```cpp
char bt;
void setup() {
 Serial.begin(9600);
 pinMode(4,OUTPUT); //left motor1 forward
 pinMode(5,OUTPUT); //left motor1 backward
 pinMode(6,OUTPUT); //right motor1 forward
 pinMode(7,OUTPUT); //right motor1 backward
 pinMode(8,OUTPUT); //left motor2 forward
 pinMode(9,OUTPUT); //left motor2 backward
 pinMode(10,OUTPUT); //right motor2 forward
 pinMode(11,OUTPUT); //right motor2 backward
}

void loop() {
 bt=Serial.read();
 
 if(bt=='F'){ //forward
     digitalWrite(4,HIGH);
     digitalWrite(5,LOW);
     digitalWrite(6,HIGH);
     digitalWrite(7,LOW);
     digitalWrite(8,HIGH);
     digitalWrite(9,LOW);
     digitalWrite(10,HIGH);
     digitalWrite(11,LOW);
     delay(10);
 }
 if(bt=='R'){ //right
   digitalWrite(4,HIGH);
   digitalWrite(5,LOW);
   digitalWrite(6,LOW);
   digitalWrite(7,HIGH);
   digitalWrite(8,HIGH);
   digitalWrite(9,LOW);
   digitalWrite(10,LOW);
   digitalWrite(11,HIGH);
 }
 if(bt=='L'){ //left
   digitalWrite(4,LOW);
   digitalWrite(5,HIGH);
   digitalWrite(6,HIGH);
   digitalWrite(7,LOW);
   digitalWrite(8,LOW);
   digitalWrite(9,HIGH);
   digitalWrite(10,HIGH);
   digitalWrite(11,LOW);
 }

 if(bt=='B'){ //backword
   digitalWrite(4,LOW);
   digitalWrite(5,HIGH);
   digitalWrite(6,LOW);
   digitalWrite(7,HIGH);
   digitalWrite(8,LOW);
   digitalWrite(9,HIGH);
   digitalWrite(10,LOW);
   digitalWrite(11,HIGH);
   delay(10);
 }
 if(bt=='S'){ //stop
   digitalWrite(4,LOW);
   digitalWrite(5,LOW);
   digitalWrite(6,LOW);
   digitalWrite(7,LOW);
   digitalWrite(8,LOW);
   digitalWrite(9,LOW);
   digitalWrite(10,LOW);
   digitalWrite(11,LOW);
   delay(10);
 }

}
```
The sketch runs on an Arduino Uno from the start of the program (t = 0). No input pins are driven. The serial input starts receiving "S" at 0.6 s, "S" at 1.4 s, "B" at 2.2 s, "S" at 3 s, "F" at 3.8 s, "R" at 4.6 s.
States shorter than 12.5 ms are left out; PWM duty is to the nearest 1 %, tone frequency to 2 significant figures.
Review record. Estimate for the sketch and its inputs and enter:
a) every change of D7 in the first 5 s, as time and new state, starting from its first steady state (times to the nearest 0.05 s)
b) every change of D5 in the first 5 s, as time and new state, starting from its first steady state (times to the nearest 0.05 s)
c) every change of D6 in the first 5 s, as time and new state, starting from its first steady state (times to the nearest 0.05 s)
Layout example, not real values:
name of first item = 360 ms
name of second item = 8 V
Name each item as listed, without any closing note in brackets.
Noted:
every change of D7 in the first 5 s, as time and new state, starting from its first steady state = 0 s low; 2.2 s high; 3 s low; 4.6 s high
every change of D5 in the first 5 s, as time and new state, starting from its first steady state = 0 s low; 2.2 s high; 3 s low
every change of D6 in the first 5 s, as time and new state, starting from its first steady state = 0 s low; 3.8 s high; 4.6 s low
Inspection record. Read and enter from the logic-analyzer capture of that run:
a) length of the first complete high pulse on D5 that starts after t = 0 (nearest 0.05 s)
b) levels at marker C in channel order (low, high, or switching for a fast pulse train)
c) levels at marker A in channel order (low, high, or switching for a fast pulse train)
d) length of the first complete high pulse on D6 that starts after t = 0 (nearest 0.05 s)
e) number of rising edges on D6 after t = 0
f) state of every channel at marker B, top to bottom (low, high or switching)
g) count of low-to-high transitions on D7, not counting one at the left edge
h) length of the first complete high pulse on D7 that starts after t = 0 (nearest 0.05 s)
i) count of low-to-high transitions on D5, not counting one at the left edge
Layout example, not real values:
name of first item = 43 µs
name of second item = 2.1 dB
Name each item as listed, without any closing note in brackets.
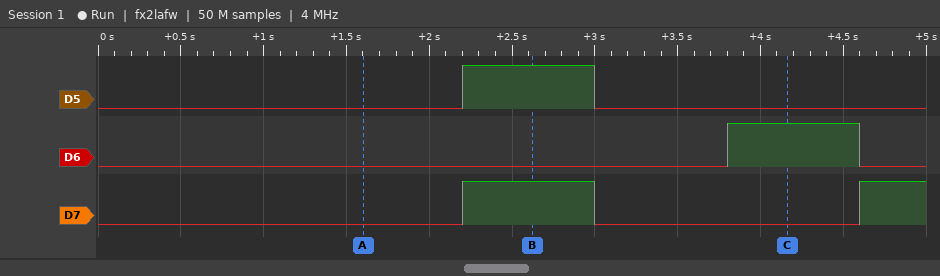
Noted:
length of the first complete high pulse on D5 that starts after t = 0 = 0.80 s
levels at marker C in channel order = D5 low, D6 high, D7 low
levels at marker A in channel order = D5 low, D6 low, D7 low
length of the first complete high pulse on D6 that starts after t = 0 = 0.80 s
number of rising edges on D6 after t = 0 = 1
state of every channel at marker B, top to bottom = D5 high, D6 low, D7 high
count of low-to-high transitions on D7, not counting one at the left edge = 2
length of the first complete high pulse on D7 that starts after t = 0 = 0.80 s
count of low-to-high transitions on D5, not counting one at the left edge = 1
